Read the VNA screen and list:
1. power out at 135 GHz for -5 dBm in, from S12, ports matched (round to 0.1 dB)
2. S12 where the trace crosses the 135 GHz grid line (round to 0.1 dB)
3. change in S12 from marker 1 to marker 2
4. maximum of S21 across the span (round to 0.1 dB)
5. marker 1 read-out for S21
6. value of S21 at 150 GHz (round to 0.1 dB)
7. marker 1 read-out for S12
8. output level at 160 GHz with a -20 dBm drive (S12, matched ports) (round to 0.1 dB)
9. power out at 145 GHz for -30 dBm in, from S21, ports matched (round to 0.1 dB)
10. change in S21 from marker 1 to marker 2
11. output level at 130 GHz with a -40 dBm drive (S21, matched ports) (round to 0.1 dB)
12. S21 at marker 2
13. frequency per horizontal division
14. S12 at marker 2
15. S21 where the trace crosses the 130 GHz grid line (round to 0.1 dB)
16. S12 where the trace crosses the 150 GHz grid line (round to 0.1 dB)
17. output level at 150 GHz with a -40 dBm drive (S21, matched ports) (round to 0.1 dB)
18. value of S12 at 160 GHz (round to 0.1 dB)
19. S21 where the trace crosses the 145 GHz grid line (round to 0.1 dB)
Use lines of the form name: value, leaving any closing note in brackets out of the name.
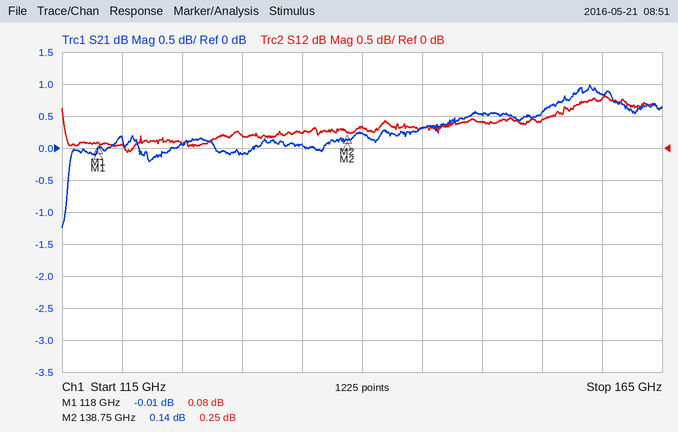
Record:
power out at 135 GHz for -5 dBm in, from S12, ports matched: -4.8 dBm
S12 where the trace crosses the 135 GHz grid line: 0.2 dB
change in S12 from marker 1 to marker 2: 0.17 dB
maximum of S21 across the span: 1.0 dB
marker 1 read-out for S21: -0.01 dB
value of S21 at 150 GHz: 0.5 dB
marker 1 read-out for S12: 0.08 dB
output level at 160 GHz with a -20 dBm drive (S12, matched ports): -19.2 dBm
power out at 145 GHz for -30 dBm in, from S21, ports matched: -29.7 dBm
change in S21 from marker 1 to marker 2: 0.15 dB
output level at 130 GHz with a -40 dBm drive (S21, matched ports): -40.1 dBm
S21 at marker 2: 0.14 dB
frequency per horizontal division: 5 GHz
S12 at marker 2: 0.25 dB
S21 where the trace crosses the 130 GHz grid line: -0.1 dB
S12 where the trace crosses the 150 GHz grid line: 0.4 dB
output level at 150 GHz with a -40 dBm drive (S21, matched ports): -39.5 dBm
value of S12 at 160 GHz: 0.8 dB
S21 where the trace crosses the 145 GHz grid line: 0.3 dB
